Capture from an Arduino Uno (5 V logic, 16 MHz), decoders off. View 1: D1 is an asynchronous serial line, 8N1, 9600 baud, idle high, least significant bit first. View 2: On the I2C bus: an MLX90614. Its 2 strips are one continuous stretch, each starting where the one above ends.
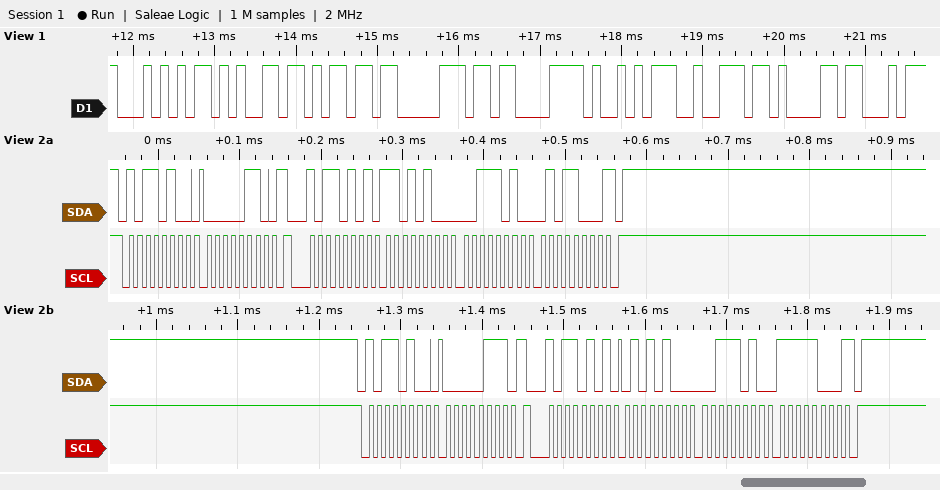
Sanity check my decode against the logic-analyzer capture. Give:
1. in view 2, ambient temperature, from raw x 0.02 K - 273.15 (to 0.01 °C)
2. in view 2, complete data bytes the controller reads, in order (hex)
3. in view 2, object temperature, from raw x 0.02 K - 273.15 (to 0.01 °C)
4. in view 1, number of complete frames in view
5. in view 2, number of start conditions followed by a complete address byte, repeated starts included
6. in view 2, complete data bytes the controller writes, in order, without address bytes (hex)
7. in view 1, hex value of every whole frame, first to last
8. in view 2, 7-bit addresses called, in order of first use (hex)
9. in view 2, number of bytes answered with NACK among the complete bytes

28.05 °C
D4 3A 58 54 3A F8
25.49 °C
8
4
06 07
54 65 6D 70 C3 A9 72 61
0x5A
2
